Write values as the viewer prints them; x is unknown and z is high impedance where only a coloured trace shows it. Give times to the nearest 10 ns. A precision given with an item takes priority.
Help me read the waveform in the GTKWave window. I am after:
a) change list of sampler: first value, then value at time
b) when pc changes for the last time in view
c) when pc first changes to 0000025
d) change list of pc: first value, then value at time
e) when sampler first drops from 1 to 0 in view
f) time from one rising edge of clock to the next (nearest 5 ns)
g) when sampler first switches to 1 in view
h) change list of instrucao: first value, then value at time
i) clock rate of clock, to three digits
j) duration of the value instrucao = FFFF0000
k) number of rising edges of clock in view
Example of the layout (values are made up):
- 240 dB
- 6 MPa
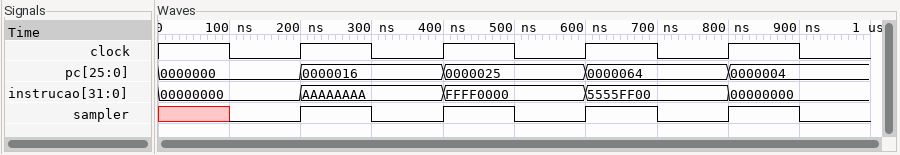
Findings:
- x, 0 at 100 ns, 1 at 200 ns, 0 at 300 ns, 1 at 400 ns, 0 at 500 ns, 1 at 600 ns, 0 at 700 ns, 1 at 800 ns, 0 at 900 ns
- 800 ns
- 400 ns
- 0000000, 0000016 at 200 ns, 0000025 at 400 ns, 0000064 at 600 ns, 0000004 at 800 ns
- 300 ns
- 200 ns
- 200 ns
- 00000000, AAAAAAAA at 200 ns, FFFF0000 at 400 ns, 5555FF00 at 600 ns, 00000000 at 800 ns
- 5.00 MHz
- 200 ns
- 4
